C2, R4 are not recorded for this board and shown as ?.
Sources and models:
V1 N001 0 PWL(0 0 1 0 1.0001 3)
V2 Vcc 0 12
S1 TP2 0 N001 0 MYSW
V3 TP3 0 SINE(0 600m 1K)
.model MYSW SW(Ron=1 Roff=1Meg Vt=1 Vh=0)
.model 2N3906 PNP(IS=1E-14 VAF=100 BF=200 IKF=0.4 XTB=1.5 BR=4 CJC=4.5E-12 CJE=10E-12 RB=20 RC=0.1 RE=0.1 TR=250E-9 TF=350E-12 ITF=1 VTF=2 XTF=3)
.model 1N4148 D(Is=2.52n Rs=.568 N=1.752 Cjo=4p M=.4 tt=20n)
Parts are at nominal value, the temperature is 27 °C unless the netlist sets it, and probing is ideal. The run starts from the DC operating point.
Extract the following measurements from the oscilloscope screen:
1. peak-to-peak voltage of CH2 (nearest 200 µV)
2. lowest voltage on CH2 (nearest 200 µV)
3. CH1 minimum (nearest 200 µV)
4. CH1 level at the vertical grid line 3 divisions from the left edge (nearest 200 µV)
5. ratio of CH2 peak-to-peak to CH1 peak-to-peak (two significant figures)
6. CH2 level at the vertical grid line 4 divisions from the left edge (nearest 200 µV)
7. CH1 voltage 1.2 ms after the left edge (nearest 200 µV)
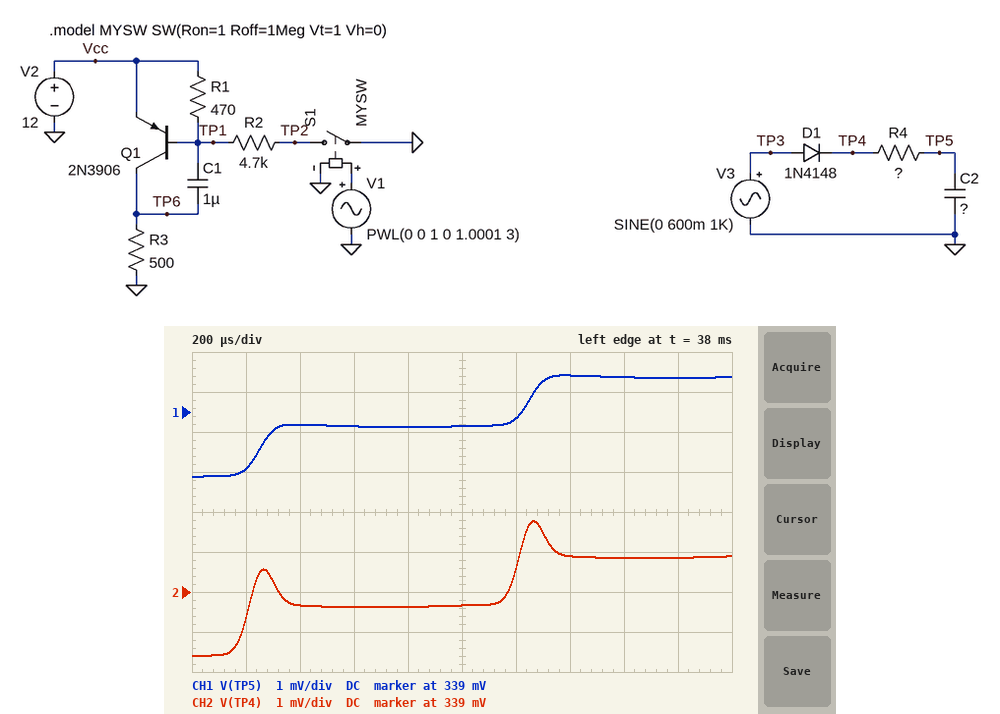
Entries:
3.4 mV
337.4 mV
337.4 mV
338.6 mV
1.3
338.6 mV
338.8 mV
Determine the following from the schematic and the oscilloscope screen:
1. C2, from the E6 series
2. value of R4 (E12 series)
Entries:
68 nF
1.8 kΩ
